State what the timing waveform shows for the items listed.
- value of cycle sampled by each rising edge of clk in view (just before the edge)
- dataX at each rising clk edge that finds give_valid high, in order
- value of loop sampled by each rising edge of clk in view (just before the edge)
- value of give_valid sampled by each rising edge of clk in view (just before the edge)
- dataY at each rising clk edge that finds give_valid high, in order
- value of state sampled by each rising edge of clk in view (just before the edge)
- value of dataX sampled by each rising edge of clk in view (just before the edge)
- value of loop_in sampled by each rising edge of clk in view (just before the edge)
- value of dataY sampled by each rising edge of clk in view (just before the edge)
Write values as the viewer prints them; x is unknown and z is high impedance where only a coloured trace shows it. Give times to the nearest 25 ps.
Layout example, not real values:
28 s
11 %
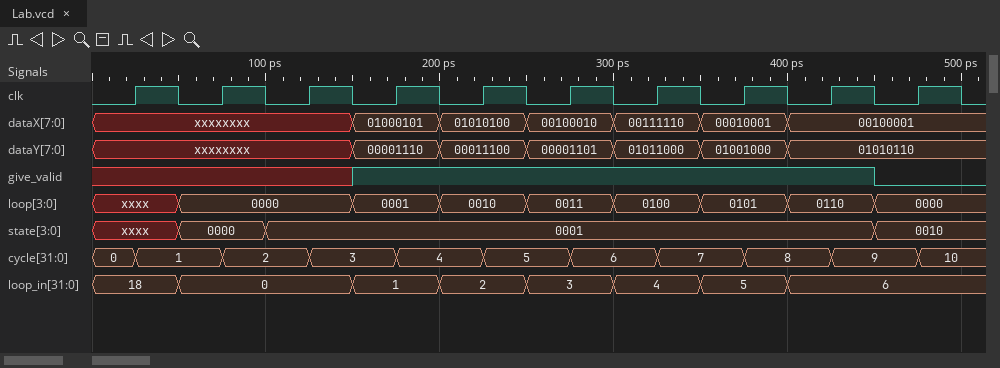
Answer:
0, 1, 2, 3, 4, 5, 6, 7, 8, 9
01000101, 01010100, 00100010, 00111110, 00010001, 00100001
xxxx, 0000, 0000, 0001, 0010, 0011, 0100, 0101, 0110, 0000
x x x 1 1 1 1 1 1 0
00001110, 00011100, 00001101, 01011000, 01001000, 01010110
xxxx, 0000, 0001, 0001, 0001, 0001, 0001, 0001, 0001, 0010
xxxxxxxx, xxxxxxxx, xxxxxxxx, 01000101, 01010100, 00100010, 00111110, 00010001, 00100001, 00100001
18, 0, 0, 1, 2, 3, 4, 5, 6, 6
xxxxxxxx, xxxxxxxx, xxxxxxxx, 00001110, 00011100, 00001101, 01011000, 01001000, 01010110, 01010110
